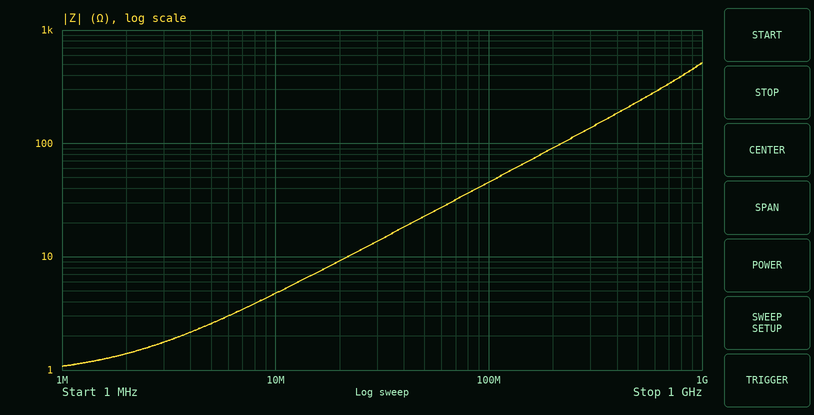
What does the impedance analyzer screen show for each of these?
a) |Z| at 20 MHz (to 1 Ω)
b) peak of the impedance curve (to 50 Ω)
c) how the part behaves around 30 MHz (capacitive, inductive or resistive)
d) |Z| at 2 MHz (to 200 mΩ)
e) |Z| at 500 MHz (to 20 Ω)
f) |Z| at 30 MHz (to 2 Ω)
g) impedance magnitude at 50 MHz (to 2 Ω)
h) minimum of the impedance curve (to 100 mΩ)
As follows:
9 Ω
500 Ω
inductive
1.4 Ω
240 Ω
14 Ω
22 Ω
1.1 Ω
